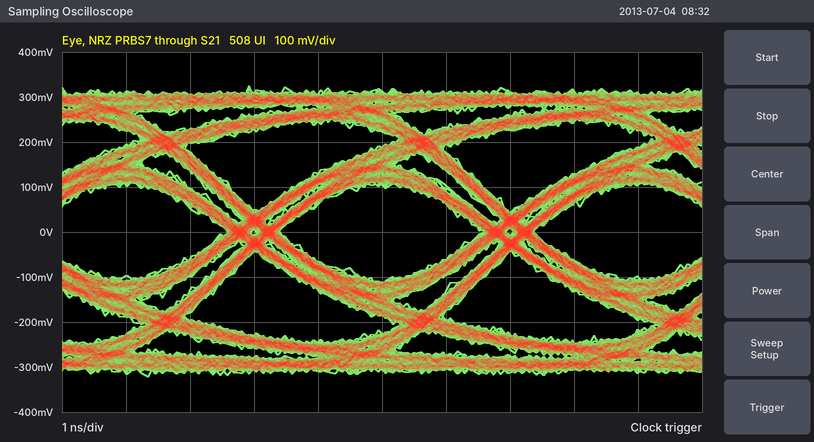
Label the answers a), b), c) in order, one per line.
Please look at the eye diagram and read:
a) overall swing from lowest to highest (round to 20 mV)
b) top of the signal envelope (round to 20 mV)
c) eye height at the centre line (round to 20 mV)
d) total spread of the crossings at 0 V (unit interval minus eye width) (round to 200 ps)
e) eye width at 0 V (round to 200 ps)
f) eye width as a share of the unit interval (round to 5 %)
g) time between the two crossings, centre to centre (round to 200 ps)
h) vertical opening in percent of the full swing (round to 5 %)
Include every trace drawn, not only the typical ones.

a) 640 mV
b) 320 mV
c) 220 mV
d) 800 ps
e) 3.2 ns
f) 80 %
g) 4.0 ns
h) 35 %
